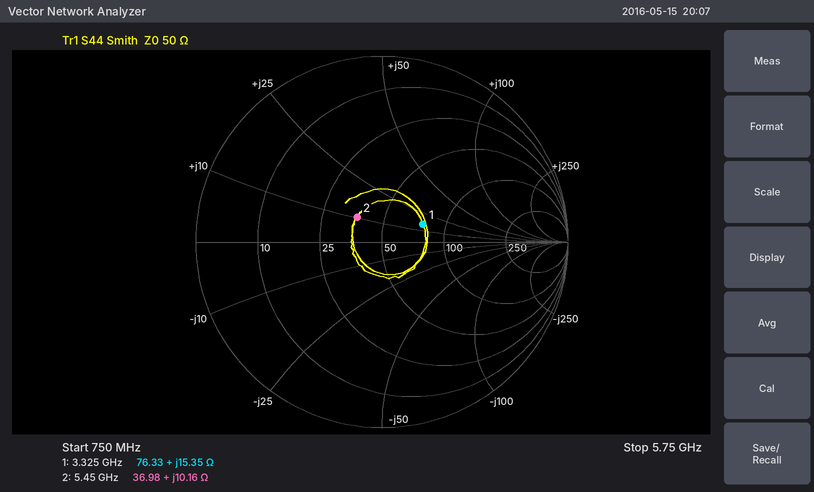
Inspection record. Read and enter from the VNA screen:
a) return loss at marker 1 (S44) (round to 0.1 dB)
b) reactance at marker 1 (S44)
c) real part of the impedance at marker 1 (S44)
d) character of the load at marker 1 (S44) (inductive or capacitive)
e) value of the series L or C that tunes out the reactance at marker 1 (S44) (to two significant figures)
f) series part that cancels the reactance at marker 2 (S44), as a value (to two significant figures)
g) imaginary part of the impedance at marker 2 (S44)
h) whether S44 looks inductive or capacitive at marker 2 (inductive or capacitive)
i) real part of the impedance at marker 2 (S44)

12.4 dB
+15.35 Ω
76.33 Ω
inductive
3.1 pF
2.9 pF
+10.16 Ω
inductive
36.98 Ω
